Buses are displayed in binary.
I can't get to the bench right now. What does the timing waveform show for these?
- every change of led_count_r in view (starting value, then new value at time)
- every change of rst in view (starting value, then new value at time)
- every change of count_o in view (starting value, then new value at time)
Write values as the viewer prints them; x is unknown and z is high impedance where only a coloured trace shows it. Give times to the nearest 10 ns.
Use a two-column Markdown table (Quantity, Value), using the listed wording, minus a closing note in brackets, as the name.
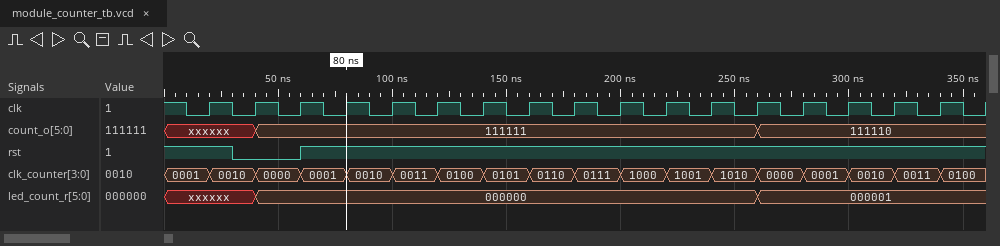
| Quantity | Value |
|---|---|
| every change of led_count_r in view | xxxxxx, 000000 at 40 ns, 000001 at 260 ns |
| every change of rst in view | 1, 0 at 30 ns, 1 at 60 ns |
| every change of count_o in view | xxxxxx, 111111 at 40 ns, 111110 at 260 ns |
